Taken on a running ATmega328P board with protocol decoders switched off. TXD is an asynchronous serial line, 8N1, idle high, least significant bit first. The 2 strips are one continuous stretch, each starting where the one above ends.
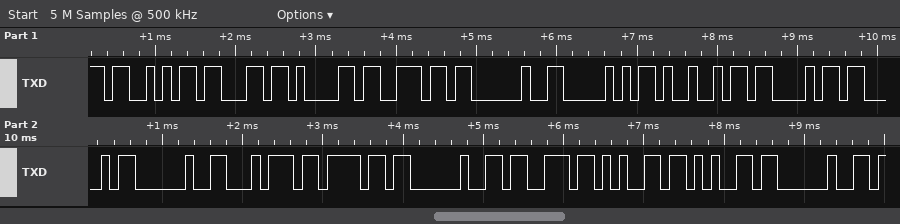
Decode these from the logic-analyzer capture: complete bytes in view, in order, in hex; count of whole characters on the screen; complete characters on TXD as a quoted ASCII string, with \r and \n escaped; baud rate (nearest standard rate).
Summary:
53 63 61 6E 20 50 49 43 43 20 74 6F 20 73 65 65 20
17
"Scan PICC to see "
9600 baud
